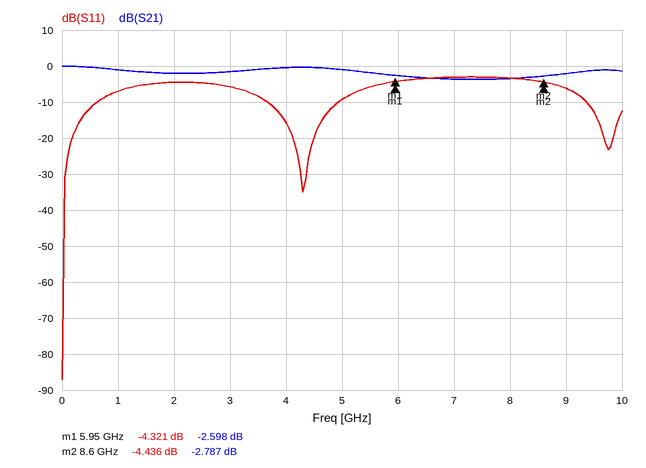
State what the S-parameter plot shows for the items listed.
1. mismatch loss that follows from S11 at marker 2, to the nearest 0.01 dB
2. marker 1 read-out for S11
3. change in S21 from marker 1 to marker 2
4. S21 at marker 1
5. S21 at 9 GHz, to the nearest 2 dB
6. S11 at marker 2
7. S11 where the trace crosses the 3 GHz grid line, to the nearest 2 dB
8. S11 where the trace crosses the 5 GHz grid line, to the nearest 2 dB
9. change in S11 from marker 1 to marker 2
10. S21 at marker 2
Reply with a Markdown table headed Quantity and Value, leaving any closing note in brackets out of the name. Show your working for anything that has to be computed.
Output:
| Quantity | Value |
|---|---|
| mismatch loss that follows from S11 at marker 2, to the nearest 0.01 dB | −10 log10(1 − 10^(-4.436/10)) ≈ 1.94 dB |
| marker 1 read-out for S11 | -4.321 dB |
| change in S21 from marker 1 to marker 2 | -2.787 − (-2.598) = -0.189 dB |
| S21 at marker 1 | -2.598 dB |
| S21 at 9 GHz, to the nearest 2 dB | -2 dB |
| S11 at marker 2 | -4.436 dB |
| S11 where the trace crosses the 3 GHz grid line, to the nearest 2 dB | -6 dB |
| S11 where the trace crosses the 5 GHz grid line, to the nearest 2 dB | -10 dB |
| change in S11 from marker 1 to marker 2 | -4.436 − (-4.321) = -0.115 dB |
| S21 at marker 2 | -2.787 dB |
